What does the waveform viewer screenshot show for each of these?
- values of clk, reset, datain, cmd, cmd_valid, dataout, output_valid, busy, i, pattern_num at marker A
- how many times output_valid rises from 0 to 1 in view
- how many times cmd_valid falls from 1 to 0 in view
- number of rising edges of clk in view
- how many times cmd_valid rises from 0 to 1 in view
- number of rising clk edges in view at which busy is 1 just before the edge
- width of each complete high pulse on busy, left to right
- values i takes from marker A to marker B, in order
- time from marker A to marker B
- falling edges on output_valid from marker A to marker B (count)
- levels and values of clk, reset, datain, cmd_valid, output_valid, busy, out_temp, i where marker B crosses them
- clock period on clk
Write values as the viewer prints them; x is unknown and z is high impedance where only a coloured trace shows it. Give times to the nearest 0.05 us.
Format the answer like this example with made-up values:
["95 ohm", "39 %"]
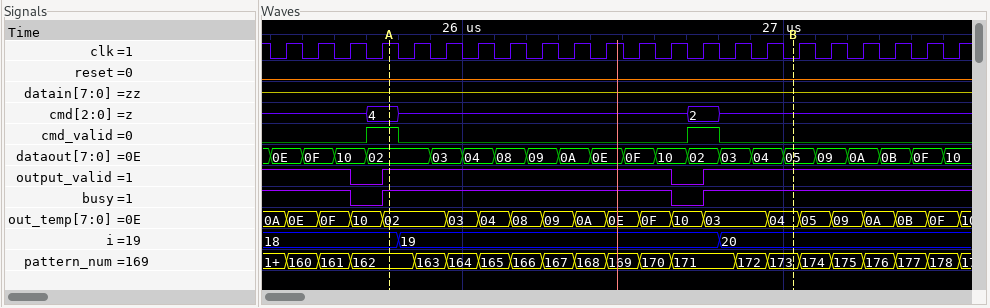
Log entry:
["clk=1, reset=0, datain=z, cmd=4, cmd_valid=1, dataout=02, output_valid=1, busy=1, i=18, pattern_num=162", "2", "2", "22", "2", "20", "0.9 us", "18, 19, 20", "1.25 us", "1", "clk=0, reset=0, datain=z, cmd_valid=0, output_valid=1, busy=1, out_temp=04, i=20", "0.1 us"]
